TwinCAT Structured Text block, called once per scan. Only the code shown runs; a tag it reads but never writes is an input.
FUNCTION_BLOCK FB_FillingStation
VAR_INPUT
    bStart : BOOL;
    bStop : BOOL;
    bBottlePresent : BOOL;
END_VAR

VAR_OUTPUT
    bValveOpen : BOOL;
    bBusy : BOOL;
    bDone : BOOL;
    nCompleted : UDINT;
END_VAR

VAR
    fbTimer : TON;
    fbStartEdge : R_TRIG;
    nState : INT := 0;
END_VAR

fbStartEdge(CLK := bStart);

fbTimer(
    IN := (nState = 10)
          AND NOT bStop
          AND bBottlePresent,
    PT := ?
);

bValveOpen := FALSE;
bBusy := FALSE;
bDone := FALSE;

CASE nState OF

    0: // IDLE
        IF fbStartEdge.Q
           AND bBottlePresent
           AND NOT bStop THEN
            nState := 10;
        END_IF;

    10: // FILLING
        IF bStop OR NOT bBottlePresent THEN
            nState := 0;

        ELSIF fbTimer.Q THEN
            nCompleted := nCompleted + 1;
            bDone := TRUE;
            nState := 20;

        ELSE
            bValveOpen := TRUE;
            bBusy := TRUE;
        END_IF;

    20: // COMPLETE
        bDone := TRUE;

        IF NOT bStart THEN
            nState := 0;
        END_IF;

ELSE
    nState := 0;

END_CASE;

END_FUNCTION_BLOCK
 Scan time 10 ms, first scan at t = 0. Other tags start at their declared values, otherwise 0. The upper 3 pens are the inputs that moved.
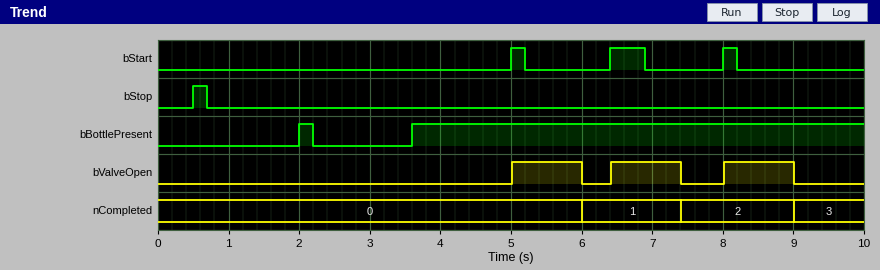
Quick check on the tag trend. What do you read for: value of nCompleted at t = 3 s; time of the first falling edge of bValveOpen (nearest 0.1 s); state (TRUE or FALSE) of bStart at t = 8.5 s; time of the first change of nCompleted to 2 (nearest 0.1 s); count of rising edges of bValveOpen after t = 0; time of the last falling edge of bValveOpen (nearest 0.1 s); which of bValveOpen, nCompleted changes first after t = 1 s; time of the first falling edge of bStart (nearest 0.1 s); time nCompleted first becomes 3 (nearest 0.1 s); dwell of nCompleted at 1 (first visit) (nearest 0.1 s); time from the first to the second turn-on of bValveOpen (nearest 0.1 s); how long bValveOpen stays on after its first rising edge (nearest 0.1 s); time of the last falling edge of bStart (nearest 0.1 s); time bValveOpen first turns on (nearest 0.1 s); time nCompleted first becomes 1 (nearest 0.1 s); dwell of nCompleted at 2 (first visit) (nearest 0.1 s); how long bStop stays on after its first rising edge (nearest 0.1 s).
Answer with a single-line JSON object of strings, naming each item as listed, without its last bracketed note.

{"value of nCompleted at t = 3 s": "0", "time of the first falling edge of bValveOpen": "6.0 s", "state (TRUE or FALSE) of bStart at t = 8.5 s": "FALSE", "time of the first change of nCompleted to 2": "7.4 s", "count of rising edges of bValveOpen after t = 0": "3", "time of the last falling edge of bValveOpen": "9.0 s", "which of bValveOpen, nCompleted changes first after t = 1 s": "bValveOpen", "time of the first falling edge of bStart": "5.2 s", "time nCompleted first becomes 3": "9.0 s", "dwell of nCompleted at 1 (first visit)": "1.4 s", "time from the first to the second turn-on of bValveOpen": "1.4 s", "how long bValveOpen stays on after its first rising edge": "1.0 s", "time of the last falling edge of bStart": "8.2 s", "time bValveOpen first turns on": "5.0 s", "time nCompleted first becomes 1": "6.0 s", "dwell of nCompleted at 2 (first visit)": "1.6 s", "how long bStop stays on after its first rising edge": "0.2 s"}
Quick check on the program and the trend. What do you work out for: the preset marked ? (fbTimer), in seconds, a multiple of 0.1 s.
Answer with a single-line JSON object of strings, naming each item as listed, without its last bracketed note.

{"the preset marked ? (fbTimer), in seconds, a multiple of 0.1 s": "1.0 s"}
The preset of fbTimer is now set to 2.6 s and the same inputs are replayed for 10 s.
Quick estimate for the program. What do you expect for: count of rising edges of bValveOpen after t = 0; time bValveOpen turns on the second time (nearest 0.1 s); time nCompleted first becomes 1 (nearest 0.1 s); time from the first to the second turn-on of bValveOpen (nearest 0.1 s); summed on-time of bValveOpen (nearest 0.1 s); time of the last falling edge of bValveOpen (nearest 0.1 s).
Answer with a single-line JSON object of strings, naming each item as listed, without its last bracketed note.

{"count of rising edges of bValveOpen after t = 0": "2", "time bValveOpen turns on the second time": "8.0 s", "time nCompleted first becomes 1": "7.6 s", "time from the first to the second turn-on of bValveOpen": "3.0 s", "summed on-time of bValveOpen": "4.6 s", "time of the last falling edge of bValveOpen": "7.6 s"}
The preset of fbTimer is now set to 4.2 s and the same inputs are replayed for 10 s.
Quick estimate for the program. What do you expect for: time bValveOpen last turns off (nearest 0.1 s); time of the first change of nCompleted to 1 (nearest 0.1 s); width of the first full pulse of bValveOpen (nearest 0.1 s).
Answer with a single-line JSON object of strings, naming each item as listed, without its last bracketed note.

{"time bValveOpen last turns off": "9.2 s", "time of the first change of nCompleted to 1": "9.2 s", "width of the first full pulse of bValveOpen": "4.2 s"}
